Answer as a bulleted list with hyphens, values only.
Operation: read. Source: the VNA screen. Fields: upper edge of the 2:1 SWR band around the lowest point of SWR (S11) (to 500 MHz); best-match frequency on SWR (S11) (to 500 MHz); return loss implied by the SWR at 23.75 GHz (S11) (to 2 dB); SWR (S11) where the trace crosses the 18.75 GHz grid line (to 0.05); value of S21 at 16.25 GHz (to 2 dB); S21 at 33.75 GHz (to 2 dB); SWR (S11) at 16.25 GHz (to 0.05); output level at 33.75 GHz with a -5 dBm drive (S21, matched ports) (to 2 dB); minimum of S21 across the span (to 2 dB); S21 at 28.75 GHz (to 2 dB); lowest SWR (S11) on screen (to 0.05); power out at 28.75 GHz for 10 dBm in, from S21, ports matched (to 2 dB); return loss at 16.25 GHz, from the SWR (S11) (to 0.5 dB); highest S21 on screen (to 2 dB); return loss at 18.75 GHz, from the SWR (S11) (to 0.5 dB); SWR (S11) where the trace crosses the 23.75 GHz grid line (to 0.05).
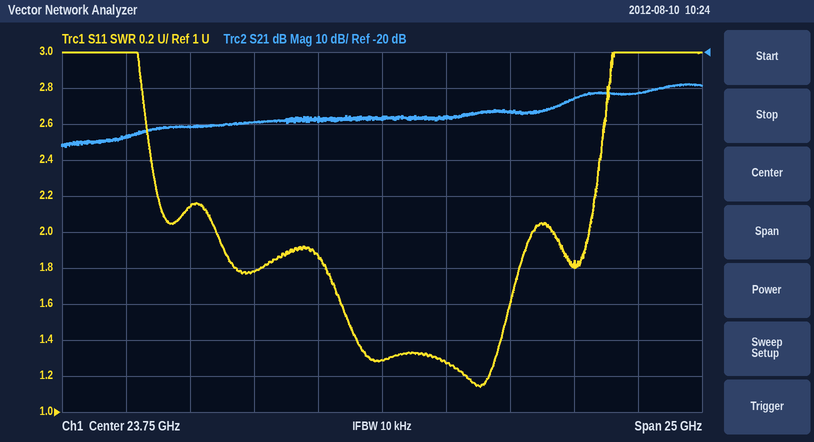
- 29.5 GHz
- 27.5 GHz
- 18 dB
- 1.80
- -40 dB
- -32 dB
- 2.15
- -36 dBm
- -46 dB
- -36 dB
- 1.15
- -26 dBm
- 9.0 dB
- -28 dB
- 11.0 dB
- 1.30
